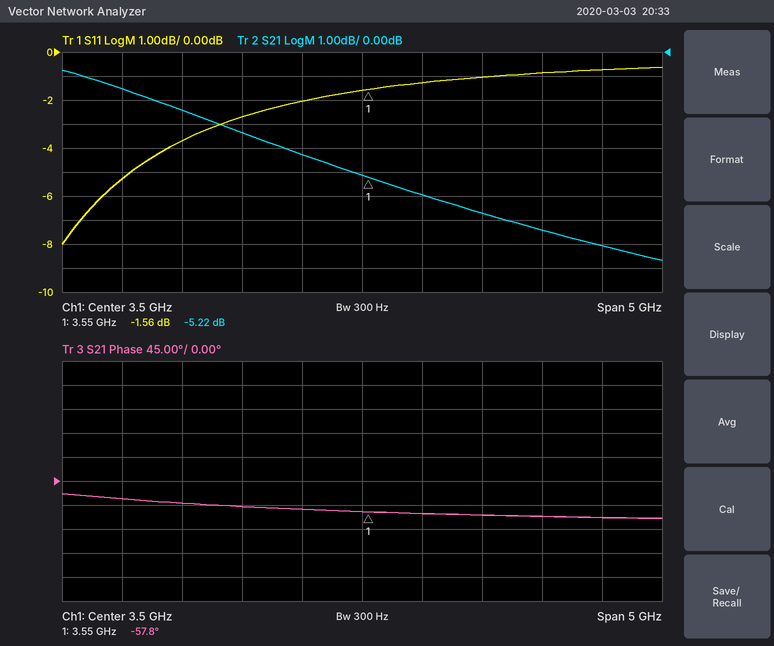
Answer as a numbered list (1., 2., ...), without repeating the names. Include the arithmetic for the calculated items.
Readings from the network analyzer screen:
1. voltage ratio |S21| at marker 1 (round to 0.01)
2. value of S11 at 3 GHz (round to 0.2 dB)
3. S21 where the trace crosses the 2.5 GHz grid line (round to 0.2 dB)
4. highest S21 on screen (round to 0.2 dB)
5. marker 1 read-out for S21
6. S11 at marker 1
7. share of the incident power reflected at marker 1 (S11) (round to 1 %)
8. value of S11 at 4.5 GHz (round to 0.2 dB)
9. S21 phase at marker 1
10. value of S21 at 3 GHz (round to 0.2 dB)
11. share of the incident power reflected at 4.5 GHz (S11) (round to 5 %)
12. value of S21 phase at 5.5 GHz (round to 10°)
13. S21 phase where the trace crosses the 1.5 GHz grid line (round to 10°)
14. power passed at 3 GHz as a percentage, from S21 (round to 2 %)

1. 10^(-5.22/20) ≈ 0.55
2. -2.0 dB
3. -3.4 dB
4. -0.8 dB
5. -5.22 dB
6. -1.56 dB
7. 10^(-1.56/10) ≈ 70 %
8. -1.0 dB
9. -57.8°
10. -4.2 dB
11. 10^(-1/10) ≈ 79.4 %, so 80 % to the nearest 5 %
12. -70°
13. -30°
14. 10^(-4.2/10) ≈ 38 %
